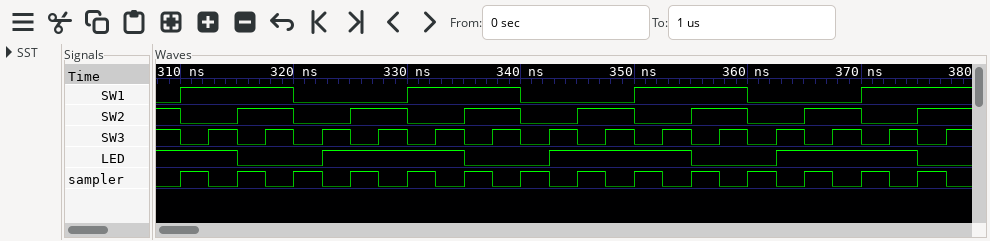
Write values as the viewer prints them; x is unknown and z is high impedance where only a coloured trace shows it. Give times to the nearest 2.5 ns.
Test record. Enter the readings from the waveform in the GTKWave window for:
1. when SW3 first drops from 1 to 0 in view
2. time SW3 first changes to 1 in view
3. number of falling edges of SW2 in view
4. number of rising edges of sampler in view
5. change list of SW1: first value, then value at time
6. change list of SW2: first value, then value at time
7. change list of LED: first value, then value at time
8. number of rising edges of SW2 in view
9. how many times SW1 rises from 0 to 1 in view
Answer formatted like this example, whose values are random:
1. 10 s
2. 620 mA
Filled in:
1. 310 ns
2. 312.5 ns
3. 7
4. 14
5. 0, 1 at 310 ns, 0 at 320 ns, 1 at 330 ns, 0 at 340 ns, 1 at 350 ns, 0 at 360 ns, 1 at 370 ns
6. 1, 0 at 310 ns, 1 at 315 ns, 0 at 320 ns, 1 at 325 ns, 0 at 330 ns, 1 at 335 ns, 0 at 340 ns, 1 at 345 ns, 0 at 350 ns, 1 at 355 ns, 0 at 360 ns, 1 at 365 ns, 0 at 370 ns, 1 at 375 ns
7. 1, 0 at 315 ns, 1 at 322.5 ns, 0 at 335 ns, 1 at 342.5 ns, 0 at 355 ns, 1 at 362.5 ns, 0 at 375 ns
8. 7
9. 4
